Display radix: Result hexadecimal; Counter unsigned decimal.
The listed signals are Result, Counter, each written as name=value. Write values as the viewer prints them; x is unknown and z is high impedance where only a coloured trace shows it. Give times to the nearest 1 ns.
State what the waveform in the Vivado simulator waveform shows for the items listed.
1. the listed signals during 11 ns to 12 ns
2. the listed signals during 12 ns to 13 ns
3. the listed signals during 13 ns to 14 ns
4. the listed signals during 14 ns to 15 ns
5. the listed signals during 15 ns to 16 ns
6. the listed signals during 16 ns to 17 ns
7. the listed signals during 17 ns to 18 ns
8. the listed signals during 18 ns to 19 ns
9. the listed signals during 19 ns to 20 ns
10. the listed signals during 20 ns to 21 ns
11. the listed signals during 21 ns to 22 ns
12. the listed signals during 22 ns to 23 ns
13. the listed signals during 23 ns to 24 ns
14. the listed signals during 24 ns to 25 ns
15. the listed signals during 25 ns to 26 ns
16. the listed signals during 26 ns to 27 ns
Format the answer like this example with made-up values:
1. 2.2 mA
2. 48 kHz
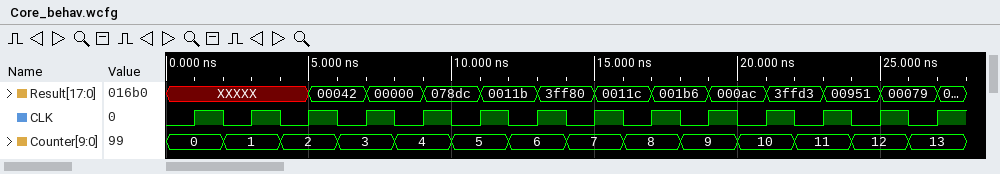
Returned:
1. Result=0011b, Counter=5
2. Result=0011b, Counter=6
3. Result=3ff80, Counter=6
4. Result=3ff80, Counter=7
5. Result=0011c, Counter=7
6. Result=0011c, Counter=8
7. Result=001b6, Counter=8
8. Result=001b6, Counter=9
9. Result=000ac, Counter=9
10. Result=000ac, Counter=10
11. Result=3ffd3, Counter=10
12. Result=3ffd3, Counter=11
13. Result=00951, Counter=11
14. Result=00951, Counter=12
15. Result=00079, Counter=12
16. Result=00079, Counter=13
